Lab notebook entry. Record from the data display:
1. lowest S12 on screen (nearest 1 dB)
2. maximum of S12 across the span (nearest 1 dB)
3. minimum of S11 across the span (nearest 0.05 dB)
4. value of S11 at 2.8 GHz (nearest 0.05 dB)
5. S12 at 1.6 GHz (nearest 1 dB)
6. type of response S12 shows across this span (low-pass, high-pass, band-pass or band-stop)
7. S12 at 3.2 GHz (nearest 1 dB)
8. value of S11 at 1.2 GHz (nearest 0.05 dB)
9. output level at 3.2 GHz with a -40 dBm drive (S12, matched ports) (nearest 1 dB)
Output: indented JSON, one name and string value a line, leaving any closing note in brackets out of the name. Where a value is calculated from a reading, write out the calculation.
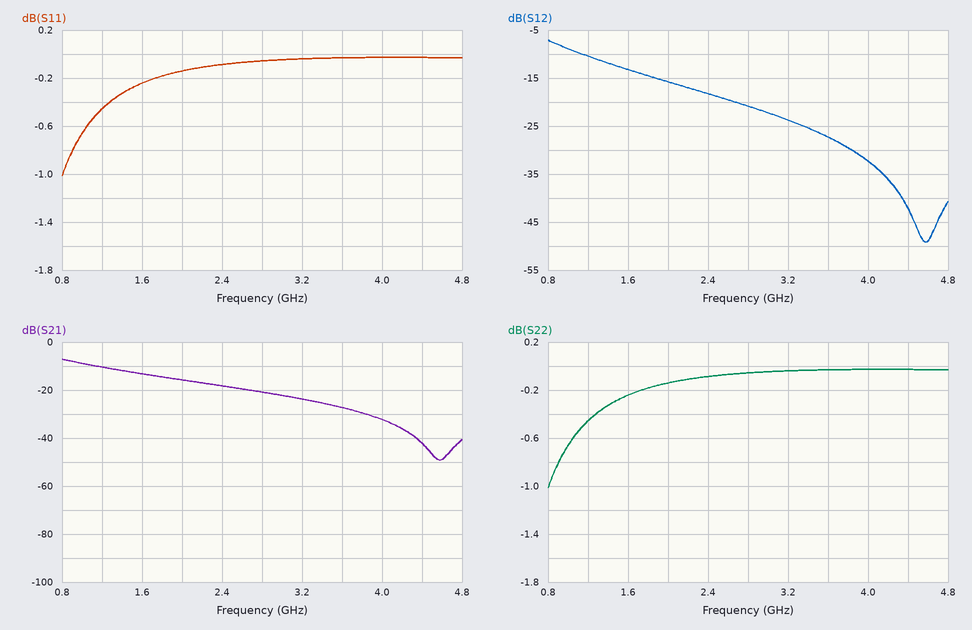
{
  "lowest S12 on screen": "-49 dB",
  "maximum of S12 across the span": "-7 dB",
  "minimum of S11 across the span": "-1.00 dB",
  "value of S11 at 2.8 GHz": "-0.05 dB",
  "S12 at 1.6 GHz": "-13 dB",
  "type of response S12 shows across this span": "low-pass",
  "S12 at 3.2 GHz": "-24 dB",
  "value of S11 at 1.2 GHz": "-0.45 dB",
  "output level at 3.2 GHz with a -40 dBm drive (S12, matched ports)": "-40 dBm + (-24 dB) = -64 dBm"
}
